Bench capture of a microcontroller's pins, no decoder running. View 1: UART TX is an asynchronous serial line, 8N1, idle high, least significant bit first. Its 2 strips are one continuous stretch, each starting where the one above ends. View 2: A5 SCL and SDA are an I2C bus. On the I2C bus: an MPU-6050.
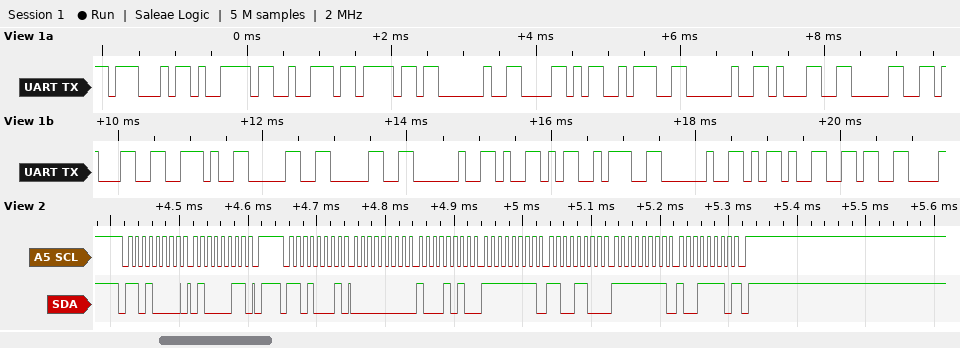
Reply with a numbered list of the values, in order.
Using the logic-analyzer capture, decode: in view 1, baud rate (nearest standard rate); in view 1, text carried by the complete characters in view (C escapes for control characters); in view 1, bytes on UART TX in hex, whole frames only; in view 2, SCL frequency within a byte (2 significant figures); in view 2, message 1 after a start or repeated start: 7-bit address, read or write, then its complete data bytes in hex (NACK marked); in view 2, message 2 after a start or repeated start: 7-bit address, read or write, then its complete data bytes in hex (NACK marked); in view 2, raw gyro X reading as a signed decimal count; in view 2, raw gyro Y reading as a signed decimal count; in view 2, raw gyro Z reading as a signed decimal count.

1. 9600 baud
2. "Gyro X: 101.00 Y: -6"
3. 47 79 72 6F 20 58 3A 20 31 30 31 2E 30 30 20 59 3A 20 2D 36
4. 100 kHz
5. 0x68 write: 43
6. 0x68 read: 00 8A FF CC FF 9E NACK
7. 138
8. -52
9. -98
